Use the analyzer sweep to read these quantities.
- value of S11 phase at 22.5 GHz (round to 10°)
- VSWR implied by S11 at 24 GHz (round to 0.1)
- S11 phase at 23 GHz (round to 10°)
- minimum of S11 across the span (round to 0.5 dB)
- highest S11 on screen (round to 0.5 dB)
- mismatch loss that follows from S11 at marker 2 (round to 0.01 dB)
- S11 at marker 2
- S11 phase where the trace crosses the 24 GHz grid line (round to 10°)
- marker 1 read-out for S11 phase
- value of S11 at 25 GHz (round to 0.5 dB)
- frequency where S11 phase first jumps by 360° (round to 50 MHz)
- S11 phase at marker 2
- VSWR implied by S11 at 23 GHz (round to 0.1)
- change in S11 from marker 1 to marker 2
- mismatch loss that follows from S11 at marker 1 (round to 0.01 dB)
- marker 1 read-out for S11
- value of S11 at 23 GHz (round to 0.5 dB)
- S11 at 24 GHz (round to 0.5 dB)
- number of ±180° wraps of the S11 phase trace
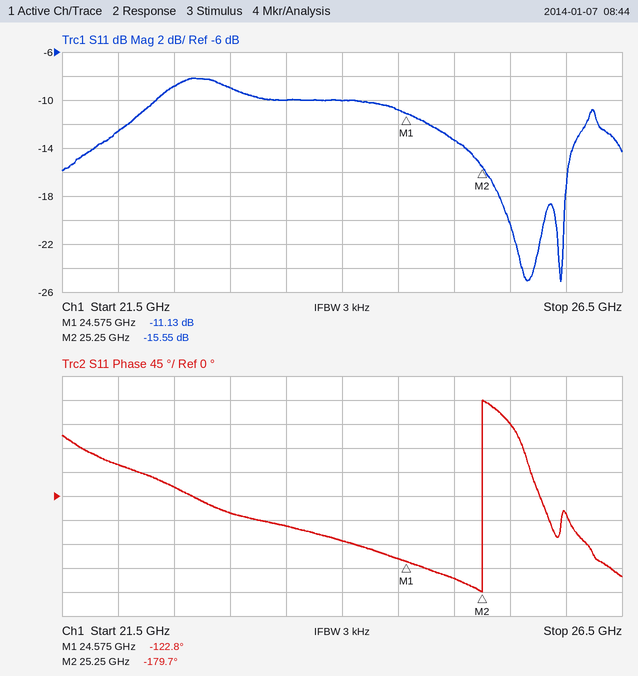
20°
1.9
-30°
-25.0 dB
-8.0 dB
0.12 dB
-15.55 dB
-80°
-122.8°
-13.5 dB
25.25 GHz
-179.7°
2.1
-4.42 dB
0.35 dB
-11.13 dB
-9.0 dB
-10.0 dB
1
